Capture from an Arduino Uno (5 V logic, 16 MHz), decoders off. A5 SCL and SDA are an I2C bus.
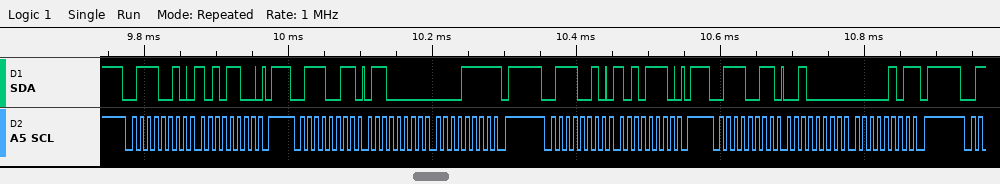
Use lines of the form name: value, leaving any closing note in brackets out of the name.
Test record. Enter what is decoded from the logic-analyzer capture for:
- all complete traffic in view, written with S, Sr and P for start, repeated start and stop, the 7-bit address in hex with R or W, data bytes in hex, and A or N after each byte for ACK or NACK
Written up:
all complete traffic in view, written with S, Sr and P for start, repeated start and stop, the 7-bit address in hex with R or W, data bytes in hex, and A or N after each byte for ACK or NACK: S 39W A AC A P S 39R A 60 A 0F N P S 39W A AE A P S 39R A 20 A 05 N P
